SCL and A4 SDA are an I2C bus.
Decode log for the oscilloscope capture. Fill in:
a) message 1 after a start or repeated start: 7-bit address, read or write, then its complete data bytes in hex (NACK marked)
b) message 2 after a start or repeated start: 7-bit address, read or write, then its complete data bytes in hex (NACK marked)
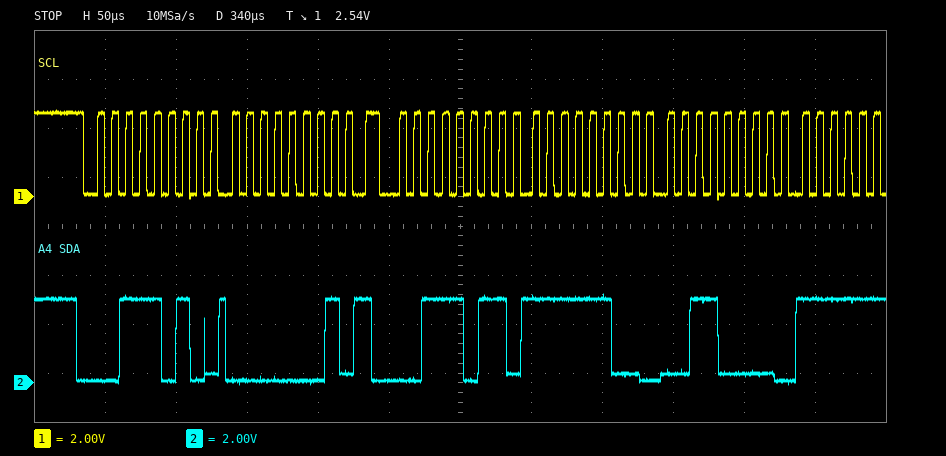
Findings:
0x1D write: 01
0x1D read: FC 30
